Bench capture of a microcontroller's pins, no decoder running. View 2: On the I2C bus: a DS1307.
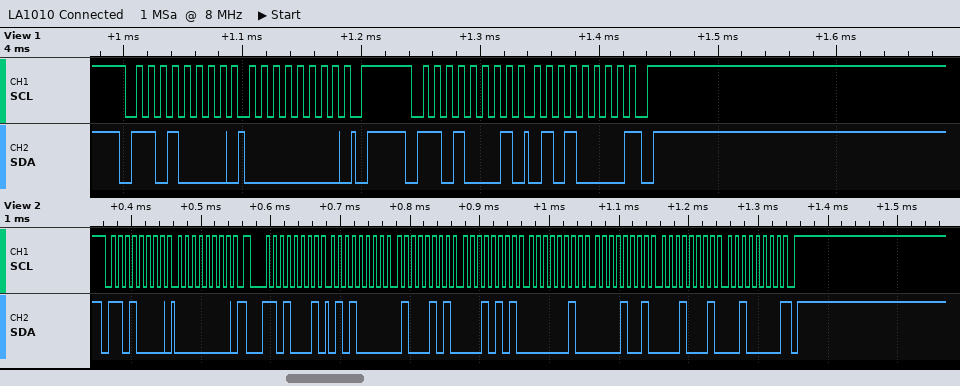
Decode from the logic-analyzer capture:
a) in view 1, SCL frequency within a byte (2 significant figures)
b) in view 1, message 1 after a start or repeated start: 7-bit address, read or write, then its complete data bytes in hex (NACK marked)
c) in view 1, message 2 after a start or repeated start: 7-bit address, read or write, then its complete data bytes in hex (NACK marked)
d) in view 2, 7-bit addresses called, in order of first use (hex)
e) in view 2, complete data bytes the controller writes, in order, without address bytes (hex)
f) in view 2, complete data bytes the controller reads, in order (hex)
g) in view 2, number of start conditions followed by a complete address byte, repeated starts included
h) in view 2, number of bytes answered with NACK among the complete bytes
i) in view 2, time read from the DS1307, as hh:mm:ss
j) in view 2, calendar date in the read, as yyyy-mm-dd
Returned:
100 kHz
0x68 write: 00
0x68 read: 50 NACK
0x68
00
50 45 15 02 09 11 20
2
1
15:45:50
2020-11-09
